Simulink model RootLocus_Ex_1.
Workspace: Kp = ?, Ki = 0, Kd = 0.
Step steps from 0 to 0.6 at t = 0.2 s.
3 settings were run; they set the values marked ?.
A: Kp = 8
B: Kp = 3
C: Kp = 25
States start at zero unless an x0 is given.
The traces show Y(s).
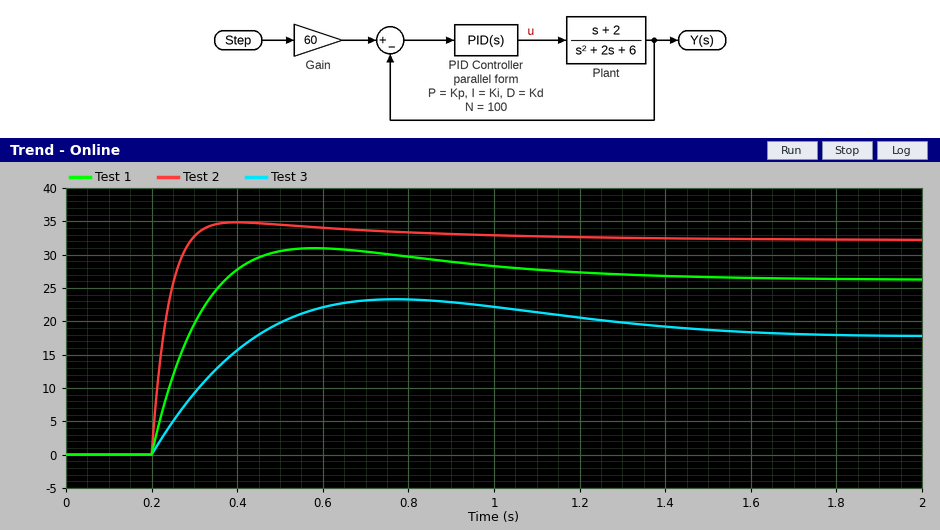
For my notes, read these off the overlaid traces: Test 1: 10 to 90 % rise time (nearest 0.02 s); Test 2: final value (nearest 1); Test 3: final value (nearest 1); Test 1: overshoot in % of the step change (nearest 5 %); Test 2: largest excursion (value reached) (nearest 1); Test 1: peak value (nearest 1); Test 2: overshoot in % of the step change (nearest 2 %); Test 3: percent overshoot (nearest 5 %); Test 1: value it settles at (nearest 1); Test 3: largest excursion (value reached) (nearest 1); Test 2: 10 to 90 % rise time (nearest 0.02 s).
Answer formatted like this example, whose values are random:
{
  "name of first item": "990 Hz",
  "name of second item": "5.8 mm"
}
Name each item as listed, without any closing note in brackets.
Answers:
{
  "Test 1: 10 to 90 % rise time": "0.12 s",
  "Test 2: final value": "32",
  "Test 3: final value": "18",
  "Test 1: overshoot in % of the step change": "20 %",
  "Test 2: largest excursion (value reached)": "35",
  "Test 1: peak value": "31",
  "Test 2: overshoot in % of the step change": "8 %",
  "Test 3: percent overshoot": "30 %",
  "Test 1: value it settles at": "26",
  "Test 3: largest excursion (value reached)": "23",
  "Test 2: 10 to 90 % rise time": "0.06 s"
}
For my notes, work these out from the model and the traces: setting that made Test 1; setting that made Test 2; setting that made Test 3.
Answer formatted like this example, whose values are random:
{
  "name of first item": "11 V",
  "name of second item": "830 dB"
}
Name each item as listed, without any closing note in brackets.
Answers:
{
  "setting that made Test 1": "A",
  "setting that made Test 2": "C",
  "setting that made Test 3": "B"
}
